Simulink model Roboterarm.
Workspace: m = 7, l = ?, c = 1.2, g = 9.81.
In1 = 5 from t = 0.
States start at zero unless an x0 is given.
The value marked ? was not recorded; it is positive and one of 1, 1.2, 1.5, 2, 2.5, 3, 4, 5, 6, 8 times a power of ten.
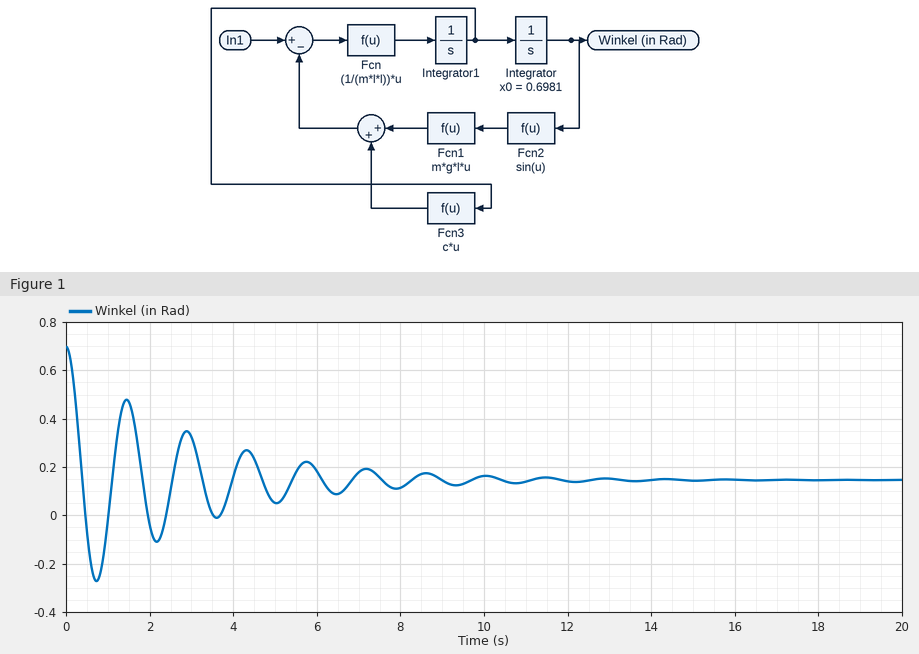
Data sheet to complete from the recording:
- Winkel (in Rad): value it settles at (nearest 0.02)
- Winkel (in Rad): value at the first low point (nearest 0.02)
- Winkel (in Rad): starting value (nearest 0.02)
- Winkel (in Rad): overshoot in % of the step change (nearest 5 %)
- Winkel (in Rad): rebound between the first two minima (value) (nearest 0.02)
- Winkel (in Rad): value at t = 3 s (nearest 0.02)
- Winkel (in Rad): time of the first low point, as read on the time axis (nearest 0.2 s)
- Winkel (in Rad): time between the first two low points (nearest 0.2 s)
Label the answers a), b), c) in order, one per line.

a) 0.14
b) -0.28
c) 0.70
d) 75 %
e) 0.48
f) 0.32
g) 0.8 s
h) 1.4 s
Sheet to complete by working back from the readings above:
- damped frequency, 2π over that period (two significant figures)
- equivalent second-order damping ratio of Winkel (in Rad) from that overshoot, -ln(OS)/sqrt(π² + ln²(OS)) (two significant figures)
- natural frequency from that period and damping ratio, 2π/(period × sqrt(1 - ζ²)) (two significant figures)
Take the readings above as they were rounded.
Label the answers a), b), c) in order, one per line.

a) 4.5 rad/s
b) 0.091
c) 4.5 rad/s
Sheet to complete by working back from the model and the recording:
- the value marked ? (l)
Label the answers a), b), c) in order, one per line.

a) 0.5
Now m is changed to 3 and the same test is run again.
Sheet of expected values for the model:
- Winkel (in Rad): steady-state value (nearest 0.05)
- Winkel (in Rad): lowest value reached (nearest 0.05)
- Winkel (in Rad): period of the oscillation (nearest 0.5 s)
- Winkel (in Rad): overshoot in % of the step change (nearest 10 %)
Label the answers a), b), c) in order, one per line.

a) 0.35
b) 0.15
c) 1.5 s
d) 50 %
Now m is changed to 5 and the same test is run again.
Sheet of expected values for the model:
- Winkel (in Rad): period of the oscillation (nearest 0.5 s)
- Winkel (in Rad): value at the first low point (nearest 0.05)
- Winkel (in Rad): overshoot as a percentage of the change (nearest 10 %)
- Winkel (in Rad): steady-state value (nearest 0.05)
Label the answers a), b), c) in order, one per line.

a) 1.5 s
b) -0.15
c) 70 %
d) 0.20
